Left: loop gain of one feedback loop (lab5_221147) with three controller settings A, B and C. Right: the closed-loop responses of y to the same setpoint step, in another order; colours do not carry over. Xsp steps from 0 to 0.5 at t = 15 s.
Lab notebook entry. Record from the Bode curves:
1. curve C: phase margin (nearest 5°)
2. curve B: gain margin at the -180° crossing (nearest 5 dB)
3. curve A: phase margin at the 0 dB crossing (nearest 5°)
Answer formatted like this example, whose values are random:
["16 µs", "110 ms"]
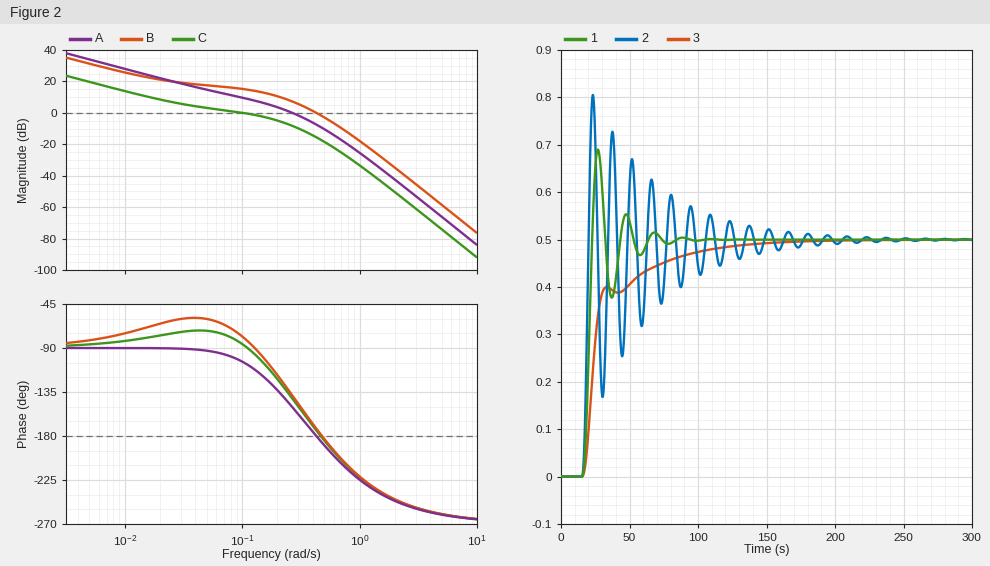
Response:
["95°", "0 dB", "30°"]
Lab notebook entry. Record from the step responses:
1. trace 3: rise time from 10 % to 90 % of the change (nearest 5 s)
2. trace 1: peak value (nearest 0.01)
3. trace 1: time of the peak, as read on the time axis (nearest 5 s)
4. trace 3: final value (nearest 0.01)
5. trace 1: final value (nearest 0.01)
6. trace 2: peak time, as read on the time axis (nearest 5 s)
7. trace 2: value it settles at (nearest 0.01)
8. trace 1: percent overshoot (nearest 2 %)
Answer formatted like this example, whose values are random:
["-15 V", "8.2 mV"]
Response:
["55 s", "0.69", "25 s", "0.50", "0.50", "25 s", "0.50", "38 %"]
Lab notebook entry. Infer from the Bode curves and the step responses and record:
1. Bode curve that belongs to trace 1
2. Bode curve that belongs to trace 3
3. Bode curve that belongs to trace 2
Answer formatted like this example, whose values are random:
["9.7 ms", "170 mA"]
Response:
["A", "C", "B"]
